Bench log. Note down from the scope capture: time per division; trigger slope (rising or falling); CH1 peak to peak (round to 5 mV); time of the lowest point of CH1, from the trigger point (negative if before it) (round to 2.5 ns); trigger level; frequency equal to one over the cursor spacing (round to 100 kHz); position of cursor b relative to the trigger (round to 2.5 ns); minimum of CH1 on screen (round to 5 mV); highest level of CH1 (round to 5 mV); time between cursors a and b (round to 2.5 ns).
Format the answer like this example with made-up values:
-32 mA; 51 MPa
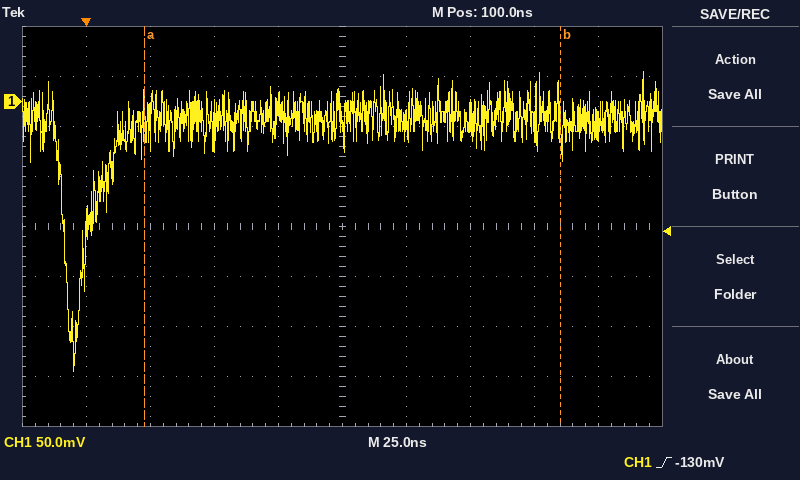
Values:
25 ns; rising; 300 mV; -5.0 ns; -130 mV; 6.2 MHz; +185.0 ns; -270 mV; 30 mV; 162.5 ns
